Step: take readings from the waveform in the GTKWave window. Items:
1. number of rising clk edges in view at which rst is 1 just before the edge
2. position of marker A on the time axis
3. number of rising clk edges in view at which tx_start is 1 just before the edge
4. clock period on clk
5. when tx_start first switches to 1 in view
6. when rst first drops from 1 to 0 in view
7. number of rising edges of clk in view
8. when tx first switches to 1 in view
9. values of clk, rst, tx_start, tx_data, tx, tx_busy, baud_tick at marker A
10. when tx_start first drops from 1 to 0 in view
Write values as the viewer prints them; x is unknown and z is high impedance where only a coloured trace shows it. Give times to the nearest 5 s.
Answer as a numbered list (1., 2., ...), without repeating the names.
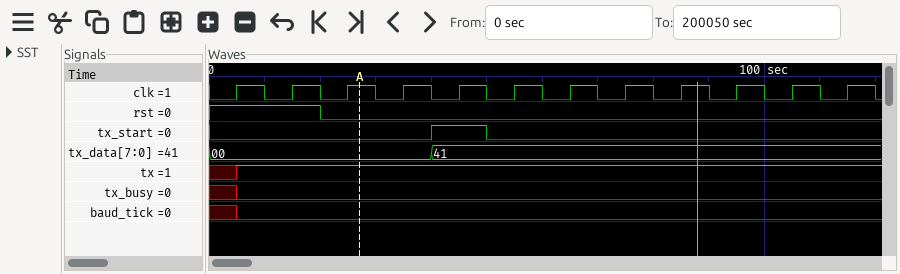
1. 2
2. 25 s
3. 1
4. 10 s
5. 40 s
6. 20 s
7. 12
8. 5 s
9. clk=1, rst=0, tx_start=0, tx_data=00, tx=1, tx_busy=0, baud_tick=0
10. 50 s
